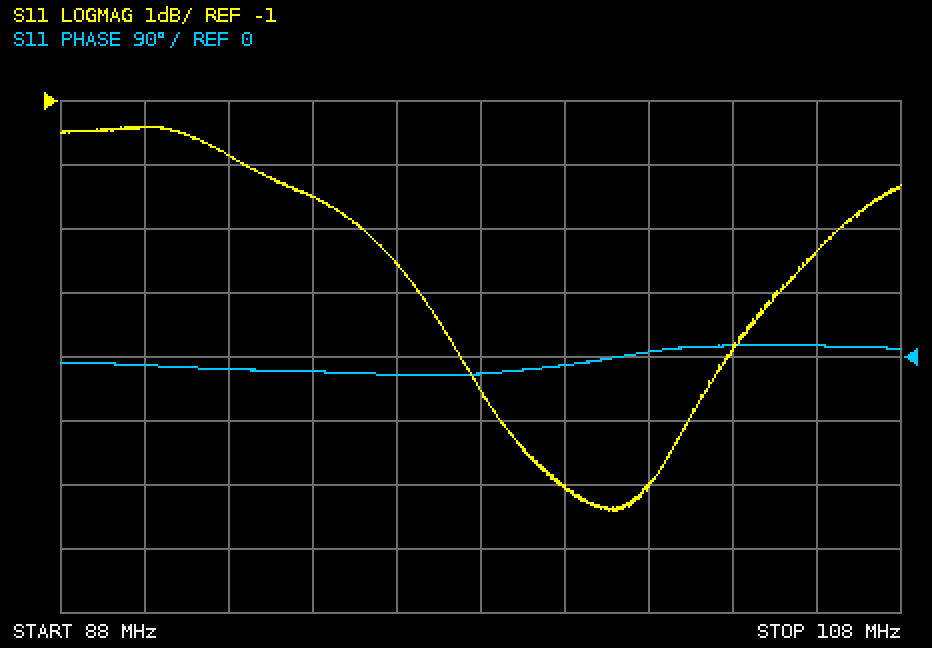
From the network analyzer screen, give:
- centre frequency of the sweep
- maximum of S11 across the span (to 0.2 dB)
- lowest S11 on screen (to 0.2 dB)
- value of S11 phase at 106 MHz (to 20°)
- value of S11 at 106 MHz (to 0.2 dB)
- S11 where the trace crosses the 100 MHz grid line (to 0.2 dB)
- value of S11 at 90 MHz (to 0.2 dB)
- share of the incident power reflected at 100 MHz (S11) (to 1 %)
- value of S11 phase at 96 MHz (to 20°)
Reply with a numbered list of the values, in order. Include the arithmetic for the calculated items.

1. 98 MHz
2. -1.4 dB
3. -7.4 dB
4. 20°
5. -3.4 dB
6. -7.0 dB
7. -1.4 dB
8. 10^(-7/10) ≈ 20 %
9. -20°
